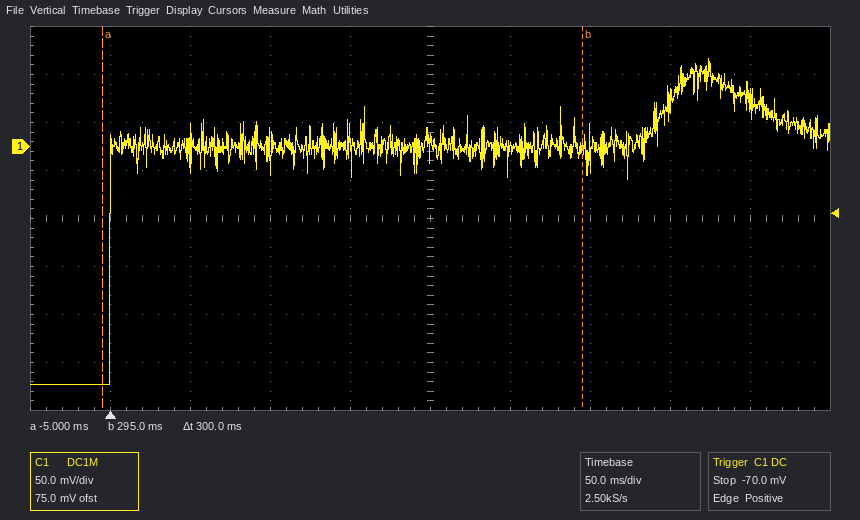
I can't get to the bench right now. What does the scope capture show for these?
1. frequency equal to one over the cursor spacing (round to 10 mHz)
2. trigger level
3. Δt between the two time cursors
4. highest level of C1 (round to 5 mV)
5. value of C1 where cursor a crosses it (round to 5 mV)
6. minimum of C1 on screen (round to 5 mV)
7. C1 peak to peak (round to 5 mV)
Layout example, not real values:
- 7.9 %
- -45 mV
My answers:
- 3.33 Hz
- -70.0 mV
- 300 ms
- 90 mV
- -250 mV
- -250 mV
- 340 mV
